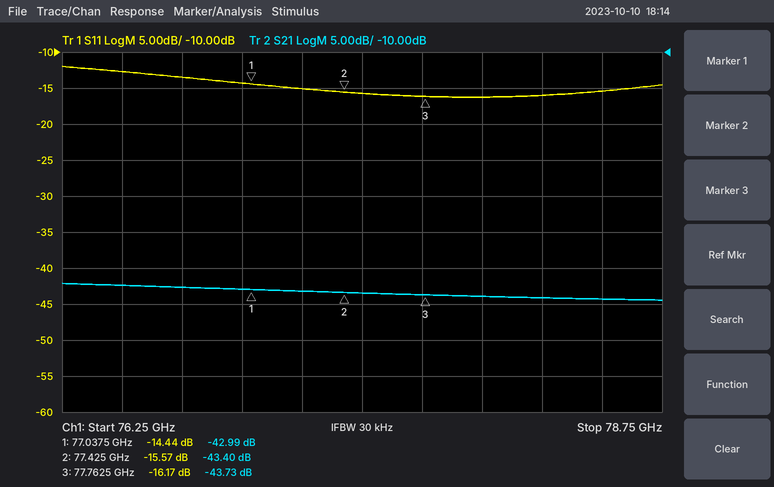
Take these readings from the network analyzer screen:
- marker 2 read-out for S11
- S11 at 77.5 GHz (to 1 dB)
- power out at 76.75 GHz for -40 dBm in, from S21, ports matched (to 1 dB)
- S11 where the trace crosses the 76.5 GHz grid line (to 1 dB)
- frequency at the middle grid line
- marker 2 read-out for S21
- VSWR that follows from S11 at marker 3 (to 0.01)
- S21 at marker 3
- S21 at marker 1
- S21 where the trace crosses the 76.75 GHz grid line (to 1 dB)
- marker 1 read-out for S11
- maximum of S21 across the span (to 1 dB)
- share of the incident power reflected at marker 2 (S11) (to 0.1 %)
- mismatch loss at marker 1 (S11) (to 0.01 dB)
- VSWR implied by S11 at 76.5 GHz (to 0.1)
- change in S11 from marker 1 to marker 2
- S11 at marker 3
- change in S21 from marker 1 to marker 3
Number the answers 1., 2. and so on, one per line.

1. -15.57 dB
2. -16 dB
3. -83 dBm
4. -13 dB
5. 77.5 GHz
6. -43.40 dB
7. 1.37
8. -43.73 dB
9. -42.99 dB
10. -43 dB
11. -14.44 dB
12. -42 dB
13. 2.8 %
14. 0.16 dB
15. 1.6
16. -1.13 dB
17. -16.17 dB
18. -0.74 dB
